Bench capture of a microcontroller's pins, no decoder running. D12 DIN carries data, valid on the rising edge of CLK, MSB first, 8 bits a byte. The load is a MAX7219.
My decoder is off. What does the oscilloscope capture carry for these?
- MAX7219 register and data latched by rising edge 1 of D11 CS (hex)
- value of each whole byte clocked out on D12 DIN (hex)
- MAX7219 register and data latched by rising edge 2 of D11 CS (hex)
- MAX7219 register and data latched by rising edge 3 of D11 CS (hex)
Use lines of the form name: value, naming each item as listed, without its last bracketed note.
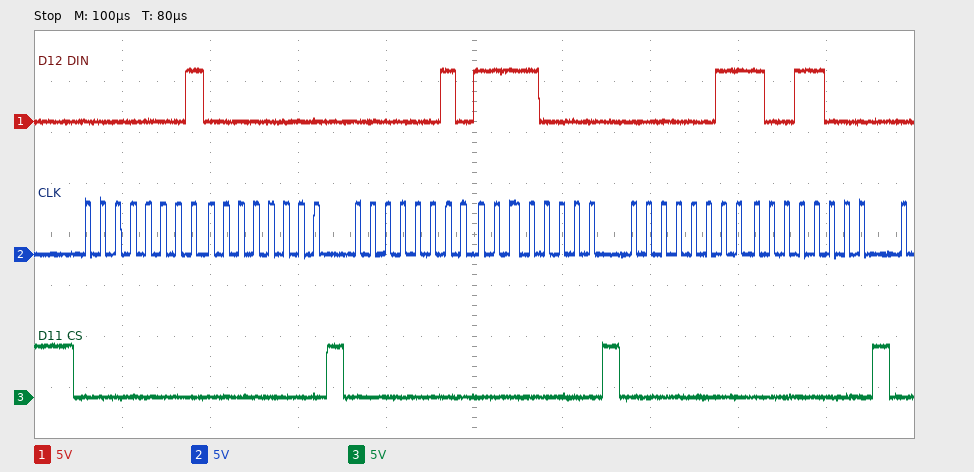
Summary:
MAX7219 register and data latched by rising edge 1 of D11 CS: register 0x1, data 0x00
value of each whole byte clocked out on D12 DIN: 01 00 02 F0 03 98
MAX7219 register and data latched by rising edge 2 of D11 CS: register 0x2, data 0xF0
MAX7219 register and data latched by rising edge 3 of D11 CS: register 0x3, data 0x98
